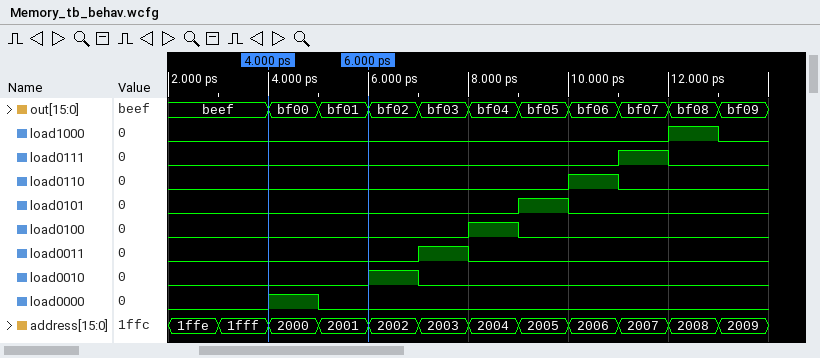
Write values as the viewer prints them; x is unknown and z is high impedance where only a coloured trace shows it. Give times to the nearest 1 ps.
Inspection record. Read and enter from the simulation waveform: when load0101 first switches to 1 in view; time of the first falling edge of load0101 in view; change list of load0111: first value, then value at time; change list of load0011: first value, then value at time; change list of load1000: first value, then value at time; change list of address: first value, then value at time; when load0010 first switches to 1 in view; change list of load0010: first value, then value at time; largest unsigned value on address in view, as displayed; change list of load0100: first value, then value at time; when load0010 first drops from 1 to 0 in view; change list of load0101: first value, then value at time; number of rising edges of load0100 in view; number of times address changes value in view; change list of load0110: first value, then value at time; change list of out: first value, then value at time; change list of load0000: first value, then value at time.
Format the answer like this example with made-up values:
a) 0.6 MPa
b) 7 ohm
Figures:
a) 9 ps
b) 10 ps
c) 0, 1 at 11 ps, 0 at 12 ps
d) 0, 1 at 7 ps, 0 at 8 ps
e) 0, 1 at 12 ps, 0 at 13 ps
f) 1ffe, 1fff at 3 ps, 2000 at 4 ps, 2001 at 5 ps, 2002 at 6 ps, 2003 at 7 ps, 2004 at 8 ps, 2005 at 9 ps, 2006 at 10 ps, 2007 at 11 ps, 2008 at 12 ps, 2009 at 13 ps
g) 6 ps
h) 0, 1 at 6 ps, 0 at 7 ps
i) 2009
j) 0, 1 at 8 ps, 0 at 9 ps
k) 7 ps
l) 0, 1 at 9 ps, 0 at 10 ps
m) 1
n) 11
o) 0, 1 at 10 ps, 0 at 11 ps
p) beef, bf00 at 4 ps, bf01 at 5 ps, bf02 at 6 ps, bf03 at 7 ps, bf04 at 8 ps, bf05 at 9 ps, bf06 at 10 ps, bf07 at 11 ps, bf08 at 12 ps, bf09 at 13 ps
q) 0, 1 at 4 ps, 0 at 5 ps
